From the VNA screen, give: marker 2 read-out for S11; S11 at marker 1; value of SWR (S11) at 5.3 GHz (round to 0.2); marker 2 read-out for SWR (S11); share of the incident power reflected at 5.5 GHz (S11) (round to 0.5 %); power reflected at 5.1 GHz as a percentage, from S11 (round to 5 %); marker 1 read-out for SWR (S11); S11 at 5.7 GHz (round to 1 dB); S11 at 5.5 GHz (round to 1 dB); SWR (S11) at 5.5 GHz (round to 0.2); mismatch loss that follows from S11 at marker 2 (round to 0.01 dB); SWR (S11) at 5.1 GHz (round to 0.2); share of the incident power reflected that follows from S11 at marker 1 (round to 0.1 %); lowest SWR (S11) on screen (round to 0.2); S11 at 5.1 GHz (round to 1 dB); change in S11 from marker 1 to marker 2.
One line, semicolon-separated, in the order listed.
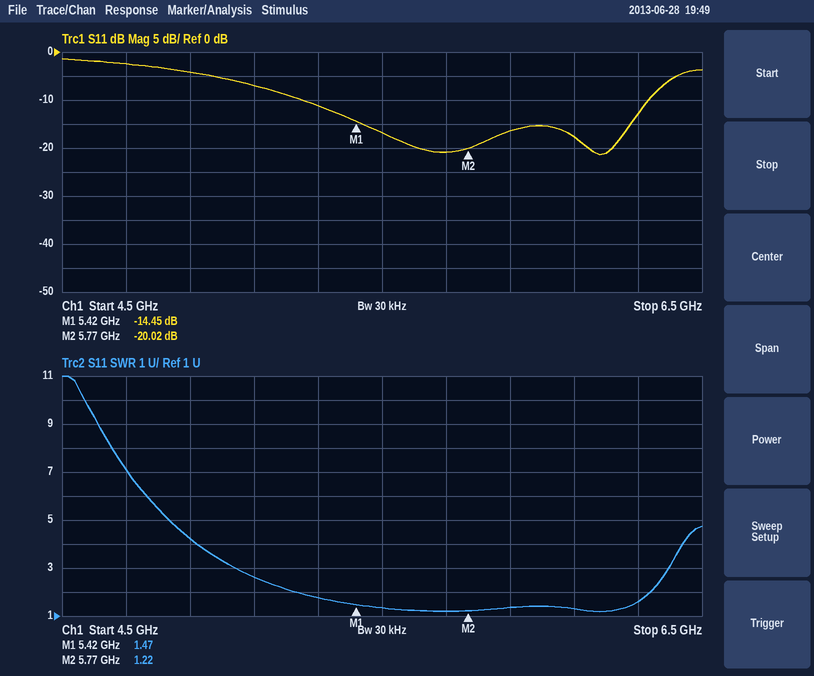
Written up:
-20.02 dB; -14.45 dB; 1.8; 1.22; 2.0 %; 20 %; 1.47; -21 dB; -17 dB; 1.4; 0.04 dB; 2.6; 3.6 %; 1.2; -7 dB; -5.57 dB
